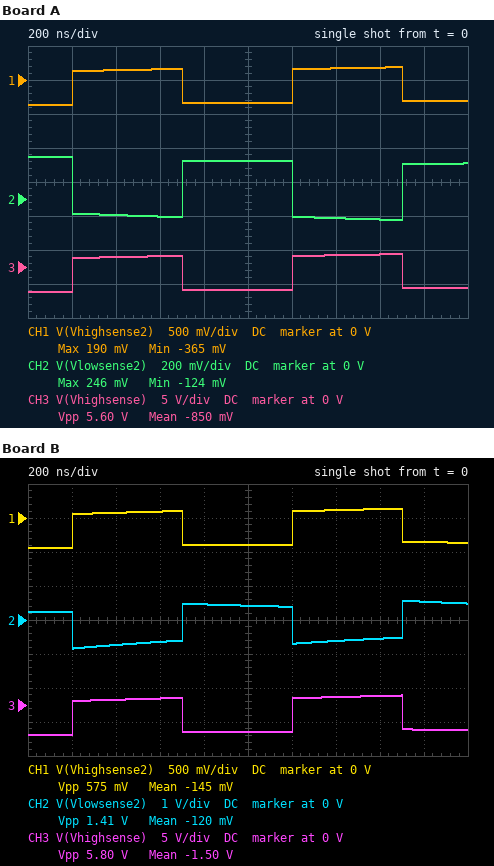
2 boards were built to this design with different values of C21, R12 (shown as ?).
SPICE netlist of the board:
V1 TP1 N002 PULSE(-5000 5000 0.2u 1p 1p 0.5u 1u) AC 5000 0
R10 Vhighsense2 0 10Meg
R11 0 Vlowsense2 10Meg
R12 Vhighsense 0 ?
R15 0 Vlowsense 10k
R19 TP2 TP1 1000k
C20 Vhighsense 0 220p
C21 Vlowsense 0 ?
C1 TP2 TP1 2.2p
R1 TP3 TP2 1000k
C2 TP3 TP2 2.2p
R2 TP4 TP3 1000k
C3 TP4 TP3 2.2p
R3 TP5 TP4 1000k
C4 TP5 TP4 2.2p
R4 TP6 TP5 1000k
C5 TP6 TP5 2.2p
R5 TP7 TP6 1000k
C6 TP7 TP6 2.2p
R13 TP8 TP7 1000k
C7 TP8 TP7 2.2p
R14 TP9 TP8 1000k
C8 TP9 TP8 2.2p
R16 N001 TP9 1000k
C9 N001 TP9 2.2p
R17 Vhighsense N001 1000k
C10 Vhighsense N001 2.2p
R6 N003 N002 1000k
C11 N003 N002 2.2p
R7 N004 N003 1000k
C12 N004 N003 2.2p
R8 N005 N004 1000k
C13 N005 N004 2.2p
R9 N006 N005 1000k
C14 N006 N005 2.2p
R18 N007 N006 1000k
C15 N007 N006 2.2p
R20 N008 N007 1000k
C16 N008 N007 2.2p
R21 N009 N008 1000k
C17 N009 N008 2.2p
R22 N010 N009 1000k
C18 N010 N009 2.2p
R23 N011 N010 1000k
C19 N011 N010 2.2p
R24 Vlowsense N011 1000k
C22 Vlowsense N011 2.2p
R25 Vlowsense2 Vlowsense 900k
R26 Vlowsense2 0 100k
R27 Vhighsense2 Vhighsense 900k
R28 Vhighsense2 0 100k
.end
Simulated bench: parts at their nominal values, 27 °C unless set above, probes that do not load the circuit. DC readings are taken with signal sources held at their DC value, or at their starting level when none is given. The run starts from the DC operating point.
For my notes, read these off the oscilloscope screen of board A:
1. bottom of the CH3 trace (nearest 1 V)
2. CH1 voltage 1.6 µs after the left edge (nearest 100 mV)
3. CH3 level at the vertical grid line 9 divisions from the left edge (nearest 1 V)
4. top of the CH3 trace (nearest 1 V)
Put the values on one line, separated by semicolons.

-4 V; 200 mV; -3 V; 2 V
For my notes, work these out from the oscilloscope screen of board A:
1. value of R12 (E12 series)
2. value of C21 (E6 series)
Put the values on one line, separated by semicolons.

15 kΩ; 330 pF
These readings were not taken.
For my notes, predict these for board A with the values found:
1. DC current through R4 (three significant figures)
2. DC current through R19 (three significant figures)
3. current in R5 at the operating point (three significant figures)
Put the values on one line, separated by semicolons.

250 µA; 250 µA; 250 µA
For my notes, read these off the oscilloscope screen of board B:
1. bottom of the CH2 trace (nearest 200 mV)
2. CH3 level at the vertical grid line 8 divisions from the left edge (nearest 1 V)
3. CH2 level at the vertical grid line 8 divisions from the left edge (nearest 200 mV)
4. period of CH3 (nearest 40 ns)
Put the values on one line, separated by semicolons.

-800 mV; 1 V; -600 mV; 1.00 µs
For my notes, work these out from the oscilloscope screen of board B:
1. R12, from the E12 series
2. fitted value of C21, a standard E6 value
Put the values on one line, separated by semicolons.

18 kΩ; 100 pF
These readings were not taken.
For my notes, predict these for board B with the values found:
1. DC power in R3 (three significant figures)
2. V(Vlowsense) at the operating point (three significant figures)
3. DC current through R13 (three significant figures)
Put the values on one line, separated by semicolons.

62.3 mW; 2.47 V; 250 µA
